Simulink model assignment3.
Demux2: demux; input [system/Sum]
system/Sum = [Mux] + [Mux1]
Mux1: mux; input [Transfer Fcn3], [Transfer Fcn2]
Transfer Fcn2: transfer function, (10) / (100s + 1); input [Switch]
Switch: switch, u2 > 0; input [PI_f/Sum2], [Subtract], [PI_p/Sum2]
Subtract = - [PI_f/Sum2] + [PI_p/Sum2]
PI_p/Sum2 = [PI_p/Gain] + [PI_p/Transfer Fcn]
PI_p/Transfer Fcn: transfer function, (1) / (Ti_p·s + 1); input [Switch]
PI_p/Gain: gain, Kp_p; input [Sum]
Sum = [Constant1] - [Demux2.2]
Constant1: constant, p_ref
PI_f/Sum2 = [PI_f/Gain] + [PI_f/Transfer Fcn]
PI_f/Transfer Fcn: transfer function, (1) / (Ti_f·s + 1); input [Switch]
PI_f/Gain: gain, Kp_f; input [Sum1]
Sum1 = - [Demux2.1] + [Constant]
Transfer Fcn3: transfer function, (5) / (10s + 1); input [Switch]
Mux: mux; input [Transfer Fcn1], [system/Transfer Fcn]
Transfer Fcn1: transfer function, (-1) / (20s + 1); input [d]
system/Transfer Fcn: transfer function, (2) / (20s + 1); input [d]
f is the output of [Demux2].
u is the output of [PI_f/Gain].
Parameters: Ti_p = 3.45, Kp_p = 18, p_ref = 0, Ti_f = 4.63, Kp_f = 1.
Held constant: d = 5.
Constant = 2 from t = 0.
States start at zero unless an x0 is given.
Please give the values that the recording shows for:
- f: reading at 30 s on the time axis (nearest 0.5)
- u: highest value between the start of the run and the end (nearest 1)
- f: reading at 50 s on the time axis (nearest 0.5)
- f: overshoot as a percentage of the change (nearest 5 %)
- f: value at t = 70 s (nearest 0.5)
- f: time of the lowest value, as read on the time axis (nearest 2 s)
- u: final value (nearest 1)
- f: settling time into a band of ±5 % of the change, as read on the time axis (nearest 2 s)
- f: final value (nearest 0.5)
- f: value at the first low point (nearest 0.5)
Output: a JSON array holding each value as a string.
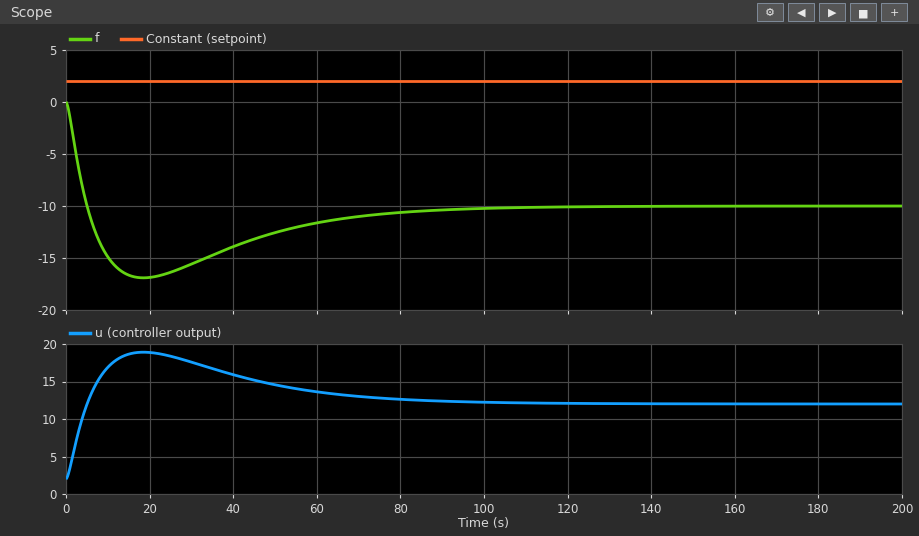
["-15.5", "19", "-12.5", "70 %", "-11.0", "18 s", "12", "84 s", "-10.0", "-17.0"]
